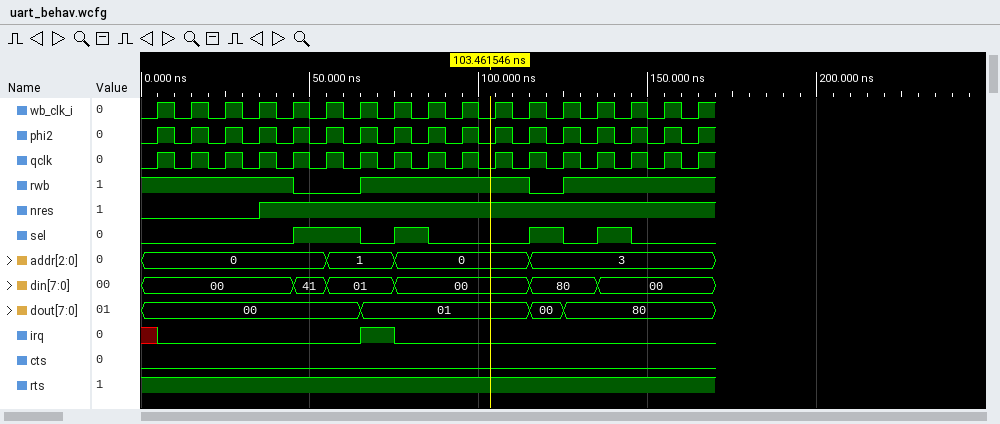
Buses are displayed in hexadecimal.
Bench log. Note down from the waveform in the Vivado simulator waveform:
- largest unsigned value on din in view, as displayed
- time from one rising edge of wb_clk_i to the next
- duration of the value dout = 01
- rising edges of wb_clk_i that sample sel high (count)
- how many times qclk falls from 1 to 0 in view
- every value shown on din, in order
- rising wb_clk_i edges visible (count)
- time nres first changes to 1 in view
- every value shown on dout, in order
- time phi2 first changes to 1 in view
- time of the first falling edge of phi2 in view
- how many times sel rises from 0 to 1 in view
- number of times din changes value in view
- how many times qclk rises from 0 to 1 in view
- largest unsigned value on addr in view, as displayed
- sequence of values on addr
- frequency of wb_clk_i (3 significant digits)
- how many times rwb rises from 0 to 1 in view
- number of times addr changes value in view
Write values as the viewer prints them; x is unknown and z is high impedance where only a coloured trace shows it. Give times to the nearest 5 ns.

80
10 ns
50 ns
5
16
00, 41, 01, 00, 80, 00
17
35 ns
00, 01, 00, 80
5 ns
10 ns
4
5
17
3
0, 1, 0, 3
100 MHz
2
3
